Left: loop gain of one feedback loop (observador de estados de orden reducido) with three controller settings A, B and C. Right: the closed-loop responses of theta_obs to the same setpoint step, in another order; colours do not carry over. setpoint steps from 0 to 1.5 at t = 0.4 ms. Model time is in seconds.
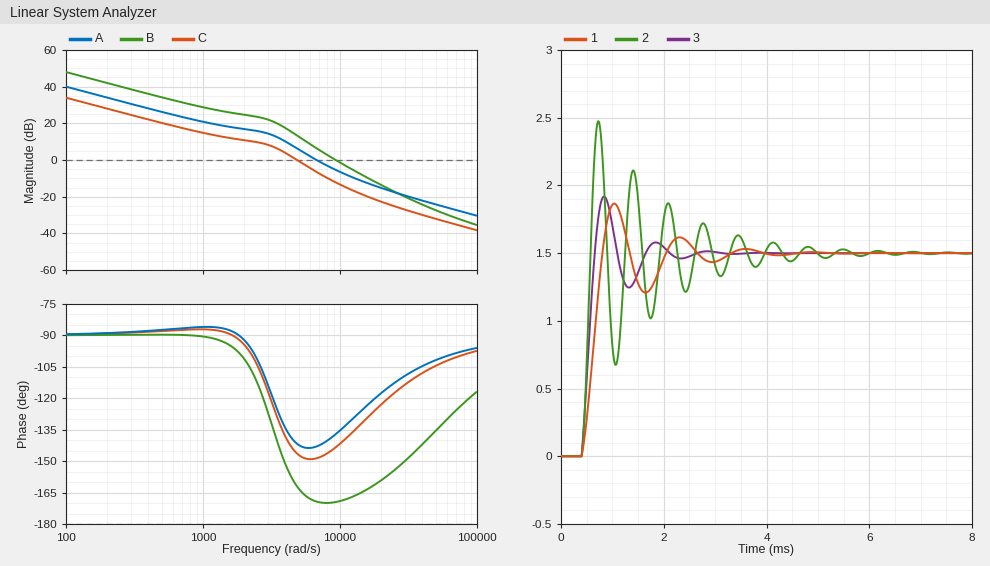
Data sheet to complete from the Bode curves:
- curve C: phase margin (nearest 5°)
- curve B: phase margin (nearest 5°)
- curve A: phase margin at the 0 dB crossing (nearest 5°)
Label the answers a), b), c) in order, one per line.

a) 35°
b) 10°
c) 35°
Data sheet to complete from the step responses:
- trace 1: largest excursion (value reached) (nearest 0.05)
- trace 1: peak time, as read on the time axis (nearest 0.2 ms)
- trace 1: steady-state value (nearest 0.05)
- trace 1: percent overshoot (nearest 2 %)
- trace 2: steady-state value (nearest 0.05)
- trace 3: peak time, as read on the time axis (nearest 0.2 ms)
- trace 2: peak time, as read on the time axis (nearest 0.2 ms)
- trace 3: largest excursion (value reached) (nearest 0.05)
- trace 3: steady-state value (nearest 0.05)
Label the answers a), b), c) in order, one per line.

a) 1.85
b) 1.0 ms
c) 1.50
d) 24 %
e) 1.50
f) 0.8 ms
g) 0.8 ms
h) 1.90
i) 1.50
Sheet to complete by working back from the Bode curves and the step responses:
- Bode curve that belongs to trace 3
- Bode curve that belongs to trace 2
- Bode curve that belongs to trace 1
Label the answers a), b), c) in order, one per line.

a) A
b) B
c) C
